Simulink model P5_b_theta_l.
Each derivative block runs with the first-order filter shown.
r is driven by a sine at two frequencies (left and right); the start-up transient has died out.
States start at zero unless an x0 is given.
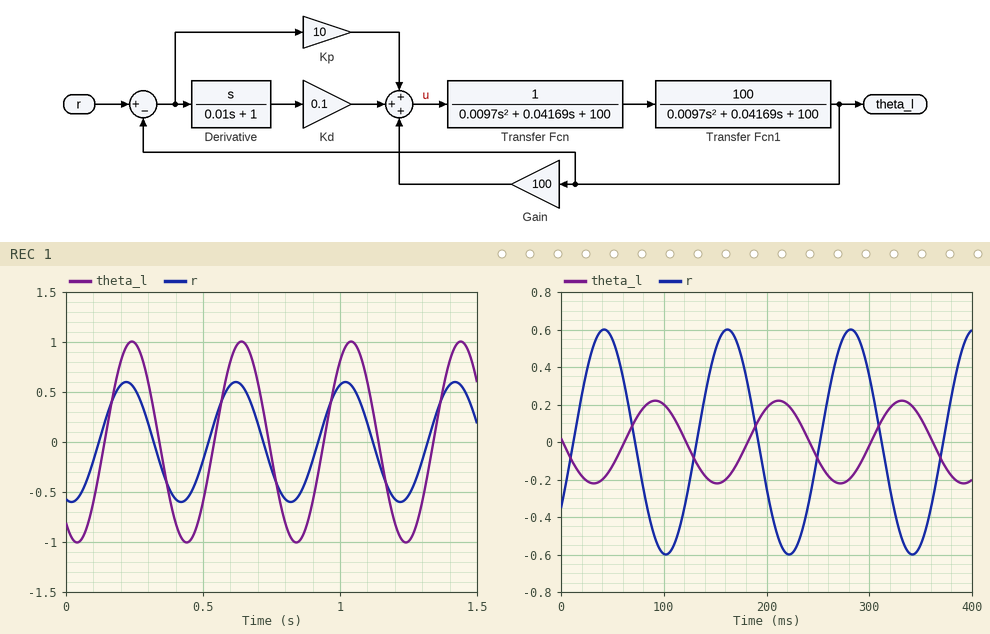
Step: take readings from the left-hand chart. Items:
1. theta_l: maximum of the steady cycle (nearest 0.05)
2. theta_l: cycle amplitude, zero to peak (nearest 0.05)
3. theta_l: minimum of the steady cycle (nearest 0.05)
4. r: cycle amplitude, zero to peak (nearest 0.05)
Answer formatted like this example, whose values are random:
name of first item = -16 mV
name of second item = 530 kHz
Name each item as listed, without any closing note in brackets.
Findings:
theta_l: maximum of the steady cycle = 1.00
theta_l: cycle amplitude, zero to peak = 1.00
theta_l: minimum of the steady cycle = -1.00
r: cycle amplitude, zero to peak = 0.60
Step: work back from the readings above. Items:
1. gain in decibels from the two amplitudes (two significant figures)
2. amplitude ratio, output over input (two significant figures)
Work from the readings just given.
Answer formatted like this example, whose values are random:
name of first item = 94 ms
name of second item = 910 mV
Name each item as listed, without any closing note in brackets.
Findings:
gain in decibels from the two amplitudes = 4.4 dB
amplitude ratio, output over input = 1.7
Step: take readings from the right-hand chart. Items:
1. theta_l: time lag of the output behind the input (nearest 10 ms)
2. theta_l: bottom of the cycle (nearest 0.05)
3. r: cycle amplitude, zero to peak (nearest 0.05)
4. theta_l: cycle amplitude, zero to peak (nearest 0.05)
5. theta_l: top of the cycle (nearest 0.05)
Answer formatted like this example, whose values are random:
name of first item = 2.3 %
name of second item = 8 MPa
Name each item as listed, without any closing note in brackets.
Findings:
theta_l: time lag of the output behind the input = 50 ms
theta_l: bottom of the cycle = -0.20
r: cycle amplitude, zero to peak = 0.60
theta_l: cycle amplitude, zero to peak = 0.20
theta_l: top of the cycle = 0.20
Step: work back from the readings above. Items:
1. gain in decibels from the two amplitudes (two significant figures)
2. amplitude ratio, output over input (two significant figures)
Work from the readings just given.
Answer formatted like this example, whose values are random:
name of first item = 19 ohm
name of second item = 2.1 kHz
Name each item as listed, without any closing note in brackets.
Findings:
gain in decibels from the two amplitudes = -9.5 dB
amplitude ratio, output over input = 0.33
